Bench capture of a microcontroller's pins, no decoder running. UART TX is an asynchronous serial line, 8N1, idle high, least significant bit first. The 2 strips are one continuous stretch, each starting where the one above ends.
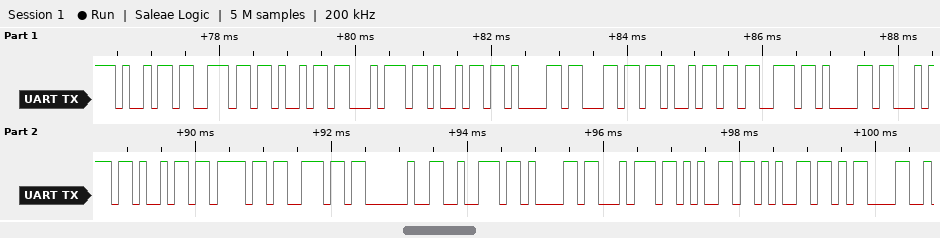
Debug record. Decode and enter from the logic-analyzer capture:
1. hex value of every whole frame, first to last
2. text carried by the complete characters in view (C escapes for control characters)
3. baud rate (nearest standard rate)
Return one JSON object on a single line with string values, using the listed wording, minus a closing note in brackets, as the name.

{"hex value of every whole frame, first to last": "0x69 0x6E 0x69 0x74 0x69 0x61 0x6C 0x69 0x73 0x61 0x74 0x69 0x6F 0x6E 0x20 0x72 0x61 0x74 0x65 0x65 0x0D", "text carried by the complete characters in view": "\"initialisation ratee\\r\"", "baud rate": "9600 baud"}
